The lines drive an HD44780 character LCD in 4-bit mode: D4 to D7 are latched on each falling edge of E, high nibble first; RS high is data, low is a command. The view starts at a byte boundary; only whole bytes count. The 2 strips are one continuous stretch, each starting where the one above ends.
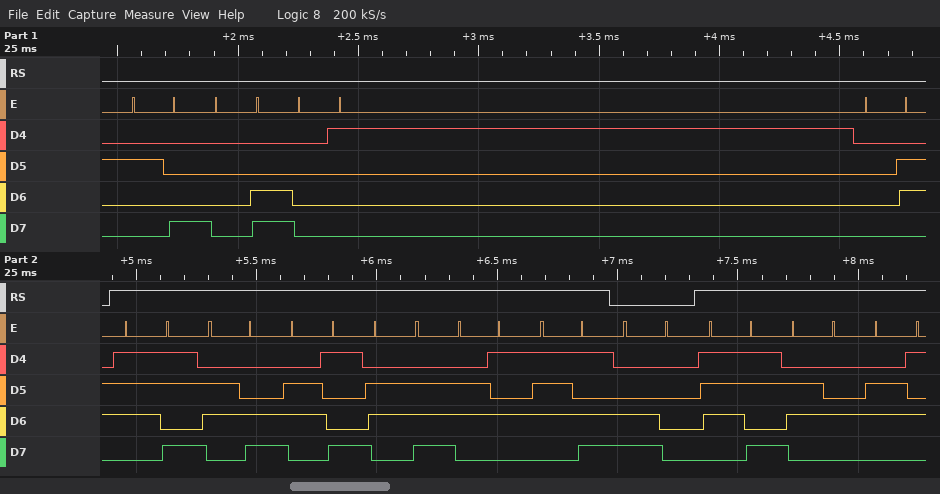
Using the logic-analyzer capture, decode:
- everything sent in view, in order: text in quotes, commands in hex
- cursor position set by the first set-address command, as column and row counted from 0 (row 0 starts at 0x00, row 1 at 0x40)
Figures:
0x28 0x0C 0x01 0x06 "{line}" 0xC0 "{de"
column 0, row 1
